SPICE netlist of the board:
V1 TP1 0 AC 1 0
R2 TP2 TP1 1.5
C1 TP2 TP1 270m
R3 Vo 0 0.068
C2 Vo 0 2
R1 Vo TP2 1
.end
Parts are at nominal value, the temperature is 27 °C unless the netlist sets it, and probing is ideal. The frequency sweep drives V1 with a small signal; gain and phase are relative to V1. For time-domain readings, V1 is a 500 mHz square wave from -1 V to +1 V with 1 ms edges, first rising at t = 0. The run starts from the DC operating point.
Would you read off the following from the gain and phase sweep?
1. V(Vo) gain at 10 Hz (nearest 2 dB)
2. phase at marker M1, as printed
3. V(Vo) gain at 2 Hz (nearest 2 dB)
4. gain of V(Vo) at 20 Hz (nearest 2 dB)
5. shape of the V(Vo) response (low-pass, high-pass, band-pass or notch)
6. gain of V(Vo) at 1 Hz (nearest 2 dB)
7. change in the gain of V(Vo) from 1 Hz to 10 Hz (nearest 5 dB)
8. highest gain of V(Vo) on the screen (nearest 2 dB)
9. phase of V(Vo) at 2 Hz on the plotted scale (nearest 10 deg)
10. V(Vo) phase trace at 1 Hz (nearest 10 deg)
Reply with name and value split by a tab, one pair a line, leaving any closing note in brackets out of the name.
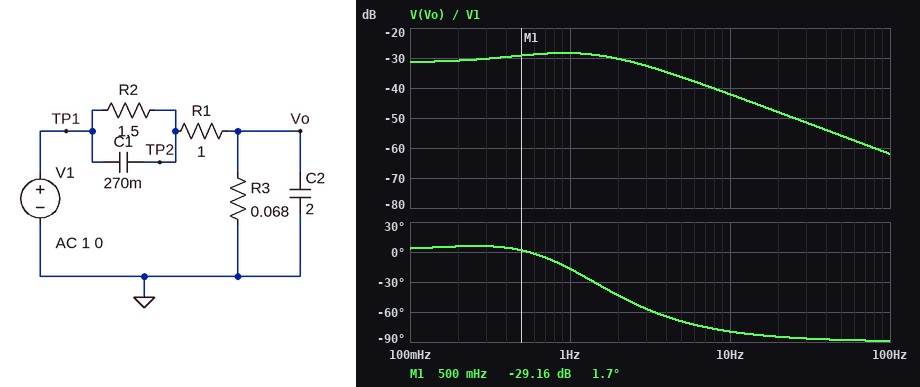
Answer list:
V(Vo) gain at 10 Hz	-42 dB
phase at marker M1, as printed	1.7 deg
V(Vo) gain at 2 Hz	-30 dB
gain of V(Vo) at 20 Hz	-48 dB
shape of the V(Vo) response	low-pass
gain of V(Vo) at 1 Hz	-28 dB
change in the gain of V(Vo) from 1 Hz to 10 Hz	-15 dB
highest gain of V(Vo) on the screen	-28 dB
phase of V(Vo) at 2 Hz on the plotted scale	-40 deg
V(Vo) phase trace at 1 Hz	-20 deg
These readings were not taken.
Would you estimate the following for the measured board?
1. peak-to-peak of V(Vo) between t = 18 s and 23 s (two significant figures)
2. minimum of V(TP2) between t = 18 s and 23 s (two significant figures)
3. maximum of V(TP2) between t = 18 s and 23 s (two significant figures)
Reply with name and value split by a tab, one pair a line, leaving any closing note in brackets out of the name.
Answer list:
peak-to-peak of V(Vo) between t = 18 s and 23 s	89 mV
minimum of V(TP2) between t = 18 s and 23 s	-1.6 V
maximum of V(TP2) between t = 18 s and 23 s	1.6 V
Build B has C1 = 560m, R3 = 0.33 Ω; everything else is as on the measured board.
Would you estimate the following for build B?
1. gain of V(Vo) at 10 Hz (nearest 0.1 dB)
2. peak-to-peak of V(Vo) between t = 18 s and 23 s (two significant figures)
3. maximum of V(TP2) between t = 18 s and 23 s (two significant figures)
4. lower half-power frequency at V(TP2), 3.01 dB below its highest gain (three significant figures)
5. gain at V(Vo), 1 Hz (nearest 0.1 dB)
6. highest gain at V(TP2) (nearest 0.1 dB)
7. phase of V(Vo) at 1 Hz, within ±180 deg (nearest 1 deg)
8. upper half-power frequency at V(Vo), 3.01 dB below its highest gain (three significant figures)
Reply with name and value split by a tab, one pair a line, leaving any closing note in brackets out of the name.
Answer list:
gain of V(Vo) at 10 Hz	-42.0 dB
peak-to-peak of V(Vo) between t = 18 s and 23 s	250 mV
maximum of V(TP2) between t = 18 s and 23 s	1.5 V
lower half-power frequency at V(TP2), 3.01 dB below its highest gain	394 mHz
gain at V(Vo), 1 Hz	-23.3 dB
highest gain at V(TP2)	0 dB
phase of V(Vo) at 1 Hz, within ±180 deg	-58 deg
upper half-power frequency at V(Vo), 3.01 dB below its highest gain	727 mHz
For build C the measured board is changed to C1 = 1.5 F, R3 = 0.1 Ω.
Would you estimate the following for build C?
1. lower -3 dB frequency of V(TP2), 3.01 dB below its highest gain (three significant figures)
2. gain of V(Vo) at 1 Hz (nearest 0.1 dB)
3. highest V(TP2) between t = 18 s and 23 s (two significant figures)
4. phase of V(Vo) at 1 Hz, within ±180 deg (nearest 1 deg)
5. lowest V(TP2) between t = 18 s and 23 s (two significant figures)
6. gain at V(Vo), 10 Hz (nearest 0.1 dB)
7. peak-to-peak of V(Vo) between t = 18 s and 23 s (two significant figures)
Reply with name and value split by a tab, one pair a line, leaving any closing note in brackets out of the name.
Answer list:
lower -3 dB frequency of V(TP2), 3.01 dB below its highest gain	136 mHz
gain of V(Vo) at 1 Hz	-24.6 dB
highest V(TP2) between t = 18 s and 23 s	1.3 V
phase of V(Vo) at 1 Hz, within ±180 deg	-43 deg
lowest V(TP2) between t = 18 s and 23 s	-1.3 V
gain at V(Vo), 10 Hz	-42.0 dB
peak-to-peak of V(Vo) between t = 18 s and 23 s	160 mV
